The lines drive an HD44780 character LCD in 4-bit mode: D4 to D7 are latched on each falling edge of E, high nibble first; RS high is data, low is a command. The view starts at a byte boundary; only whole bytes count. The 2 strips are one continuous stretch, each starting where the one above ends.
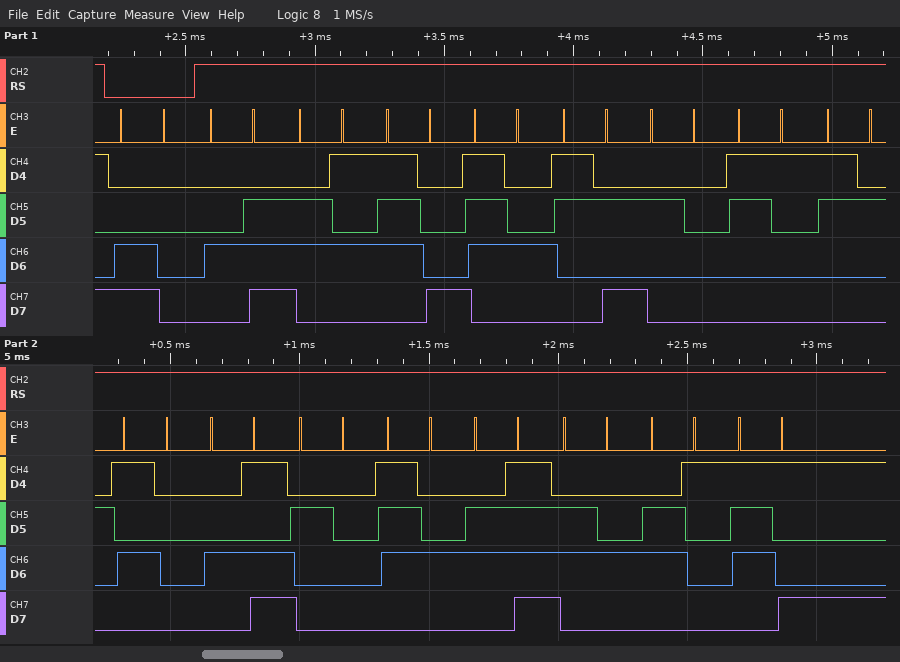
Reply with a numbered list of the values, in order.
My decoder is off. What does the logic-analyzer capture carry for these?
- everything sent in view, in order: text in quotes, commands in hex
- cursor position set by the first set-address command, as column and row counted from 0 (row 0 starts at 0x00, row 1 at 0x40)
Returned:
1. 0xC0 "Next: 12PM today"
2. column 0, row 1
